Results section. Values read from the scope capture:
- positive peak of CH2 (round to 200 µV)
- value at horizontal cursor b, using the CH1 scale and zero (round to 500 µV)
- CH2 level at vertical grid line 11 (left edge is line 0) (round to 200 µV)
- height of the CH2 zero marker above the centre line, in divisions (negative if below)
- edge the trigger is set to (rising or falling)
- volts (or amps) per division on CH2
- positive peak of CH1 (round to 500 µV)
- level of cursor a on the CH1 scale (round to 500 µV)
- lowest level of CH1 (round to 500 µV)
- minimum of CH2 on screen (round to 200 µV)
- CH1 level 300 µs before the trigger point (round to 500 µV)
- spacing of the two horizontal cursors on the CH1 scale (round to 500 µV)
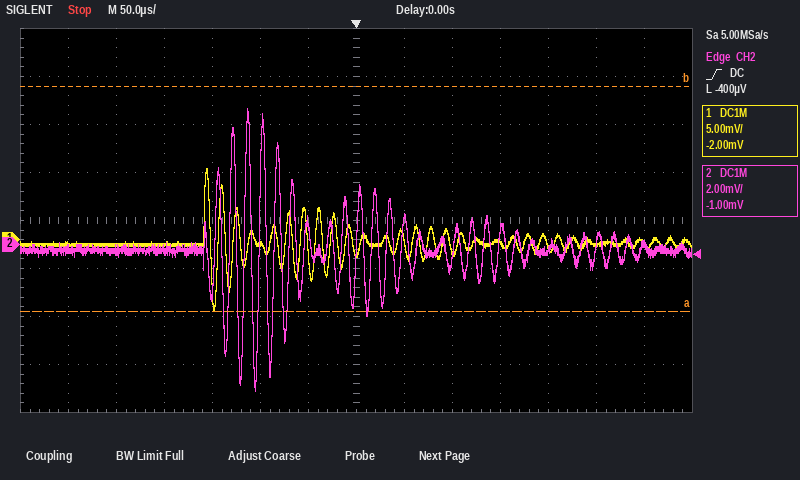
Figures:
5.6 mV
16.0 mV
-200 µV
-0.5 div
rising
2 mV
7.5 mV
-7.5 mV
-7.5 mV
-6.0 mV
-500 µV
23.5 mV
